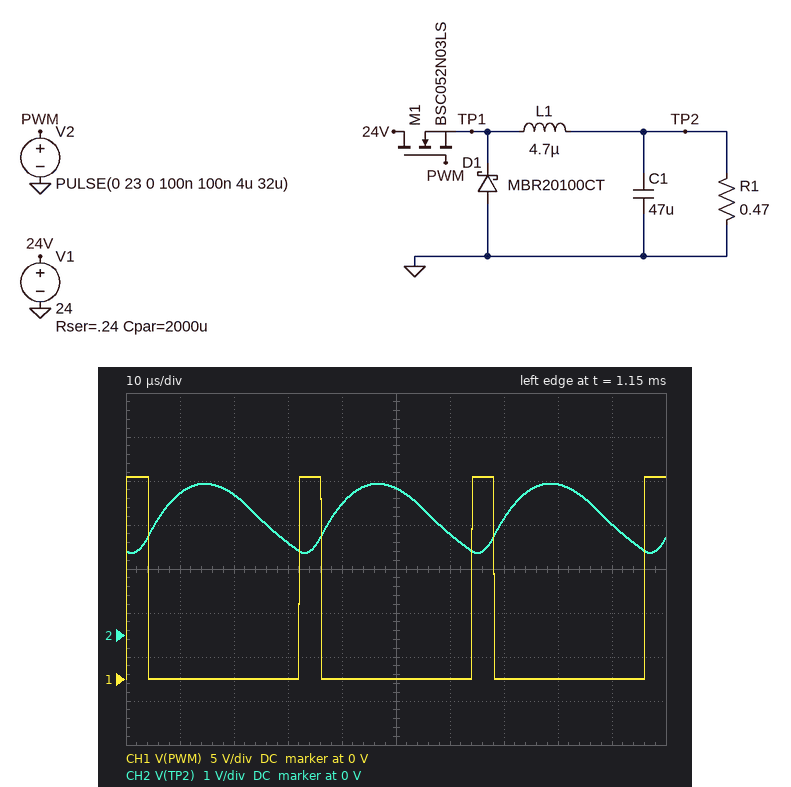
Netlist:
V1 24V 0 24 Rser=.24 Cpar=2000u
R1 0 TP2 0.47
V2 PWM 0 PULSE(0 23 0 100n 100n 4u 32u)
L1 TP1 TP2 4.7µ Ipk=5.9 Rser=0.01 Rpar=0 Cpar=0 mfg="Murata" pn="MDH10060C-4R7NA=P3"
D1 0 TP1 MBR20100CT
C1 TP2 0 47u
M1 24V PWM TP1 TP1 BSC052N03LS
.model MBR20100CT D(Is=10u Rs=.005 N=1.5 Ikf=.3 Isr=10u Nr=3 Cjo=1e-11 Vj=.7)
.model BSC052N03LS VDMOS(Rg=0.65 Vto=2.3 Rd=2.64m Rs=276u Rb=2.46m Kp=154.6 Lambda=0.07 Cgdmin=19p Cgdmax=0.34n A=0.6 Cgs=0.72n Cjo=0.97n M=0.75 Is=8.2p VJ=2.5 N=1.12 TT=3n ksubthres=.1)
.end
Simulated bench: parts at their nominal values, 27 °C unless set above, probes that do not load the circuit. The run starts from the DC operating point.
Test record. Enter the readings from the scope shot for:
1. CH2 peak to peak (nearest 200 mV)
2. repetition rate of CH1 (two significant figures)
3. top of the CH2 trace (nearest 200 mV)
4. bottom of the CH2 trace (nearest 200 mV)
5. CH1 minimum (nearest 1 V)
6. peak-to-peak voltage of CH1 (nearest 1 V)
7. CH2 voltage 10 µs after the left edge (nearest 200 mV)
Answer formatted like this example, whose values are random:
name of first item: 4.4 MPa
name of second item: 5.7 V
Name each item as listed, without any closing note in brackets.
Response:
CH2 peak to peak: 1.6 V
repetition rate of CH1: 31 kHz
top of the CH2 trace: 3.4 V
bottom of the CH2 trace: 1.8 V
CH1 minimum: 0 V
peak-to-peak voltage of CH1: 23 V
CH2 voltage 10 µs after the left edge: 3.2 V
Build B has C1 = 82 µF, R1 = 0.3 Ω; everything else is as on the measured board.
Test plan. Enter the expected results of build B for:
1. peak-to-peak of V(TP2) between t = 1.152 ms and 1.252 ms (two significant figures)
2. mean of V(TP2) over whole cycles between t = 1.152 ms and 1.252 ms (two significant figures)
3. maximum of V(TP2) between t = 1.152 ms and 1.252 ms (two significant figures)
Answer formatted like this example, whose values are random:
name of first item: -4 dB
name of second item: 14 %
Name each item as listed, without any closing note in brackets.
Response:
peak-to-peak of V(TP2) between t = 1.152 ms and 1.252 ms: 860 mV
mean of V(TP2) over whole cycles between t = 1.152 ms and 1.252 ms: 2.2 V
maximum of V(TP2) between t = 1.152 ms and 1.252 ms: 2.5 V
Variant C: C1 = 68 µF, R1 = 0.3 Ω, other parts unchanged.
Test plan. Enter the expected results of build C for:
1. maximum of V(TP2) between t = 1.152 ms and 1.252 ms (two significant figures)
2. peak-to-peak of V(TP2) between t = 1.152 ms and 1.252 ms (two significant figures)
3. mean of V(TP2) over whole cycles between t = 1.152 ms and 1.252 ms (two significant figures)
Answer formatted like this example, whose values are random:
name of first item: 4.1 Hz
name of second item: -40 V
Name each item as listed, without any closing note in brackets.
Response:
maximum of V(TP2) between t = 1.152 ms and 1.252 ms: 2.6 V
peak-to-peak of V(TP2) between t = 1.152 ms and 1.252 ms: 1.0 V
mean of V(TP2) over whole cycles between t = 1.152 ms and 1.252 ms: 2.2 V
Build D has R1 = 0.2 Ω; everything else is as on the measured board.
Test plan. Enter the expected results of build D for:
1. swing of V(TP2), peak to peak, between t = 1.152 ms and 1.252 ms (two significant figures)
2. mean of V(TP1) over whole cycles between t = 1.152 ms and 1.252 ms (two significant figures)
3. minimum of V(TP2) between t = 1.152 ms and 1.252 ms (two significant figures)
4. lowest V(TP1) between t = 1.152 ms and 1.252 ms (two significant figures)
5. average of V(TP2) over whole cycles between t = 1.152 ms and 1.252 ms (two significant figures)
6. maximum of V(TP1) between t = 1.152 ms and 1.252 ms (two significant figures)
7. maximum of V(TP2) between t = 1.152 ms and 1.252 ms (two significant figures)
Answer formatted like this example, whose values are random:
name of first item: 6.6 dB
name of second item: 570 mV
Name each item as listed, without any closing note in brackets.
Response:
swing of V(TP2), peak to peak, between t = 1.152 ms and 1.252 ms: 1.3 V
mean of V(TP1) over whole cycles between t = 1.152 ms and 1.252 ms: 2.0 V
minimum of V(TP2) between t = 1.152 ms and 1.252 ms: 1.1 V
lowest V(TP1) between t = 1.152 ms and 1.252 ms: -810 mV
average of V(TP2) over whole cycles between t = 1.152 ms and 1.252 ms: 1.9 V
maximum of V(TP1) between t = 1.152 ms and 1.252 ms: 21 V
maximum of V(TP2) between t = 1.152 ms and 1.252 ms: 2.4 V
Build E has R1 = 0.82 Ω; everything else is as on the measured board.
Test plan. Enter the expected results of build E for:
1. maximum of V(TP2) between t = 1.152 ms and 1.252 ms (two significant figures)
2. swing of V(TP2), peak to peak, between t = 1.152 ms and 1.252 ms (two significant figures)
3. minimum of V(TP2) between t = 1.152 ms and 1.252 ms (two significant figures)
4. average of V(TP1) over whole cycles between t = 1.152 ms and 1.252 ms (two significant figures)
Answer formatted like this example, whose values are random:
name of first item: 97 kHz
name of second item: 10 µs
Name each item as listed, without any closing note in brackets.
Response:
maximum of V(TP2) between t = 1.152 ms and 1.252 ms: 4.4 V
swing of V(TP2), peak to peak, between t = 1.152 ms and 1.252 ms: 1.5 V
minimum of V(TP2) between t = 1.152 ms and 1.252 ms: 2.9 V
average of V(TP1) over whole cycles between t = 1.152 ms and 1.252 ms: 3.7 V
